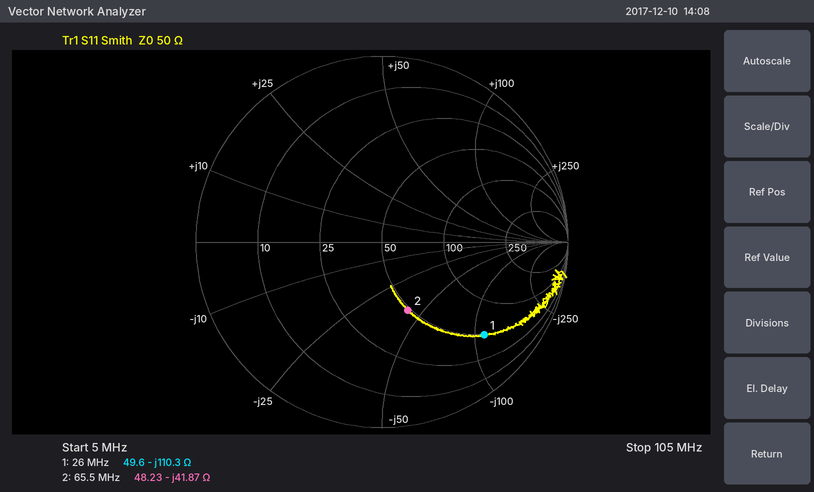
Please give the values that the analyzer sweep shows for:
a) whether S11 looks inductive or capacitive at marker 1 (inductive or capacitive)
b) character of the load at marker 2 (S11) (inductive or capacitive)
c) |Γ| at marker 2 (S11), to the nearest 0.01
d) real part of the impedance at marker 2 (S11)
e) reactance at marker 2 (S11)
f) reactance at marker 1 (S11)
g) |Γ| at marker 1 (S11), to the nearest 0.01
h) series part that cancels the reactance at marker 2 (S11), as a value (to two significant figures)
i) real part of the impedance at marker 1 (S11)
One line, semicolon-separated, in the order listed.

capacitive; capacitive; 0.39; 48.23 Ω; -41.87 Ω; -110.3 Ω; 0.74; 100 nH; 49.6 Ω
